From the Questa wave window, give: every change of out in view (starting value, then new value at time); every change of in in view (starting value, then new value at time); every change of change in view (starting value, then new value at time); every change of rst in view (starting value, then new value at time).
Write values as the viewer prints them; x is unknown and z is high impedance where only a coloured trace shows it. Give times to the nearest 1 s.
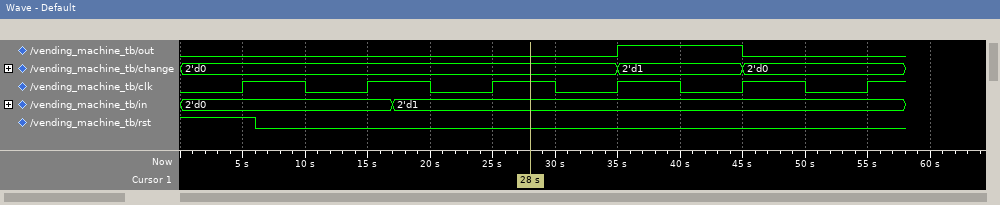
0, 1 at 35 s, 0 at 45 s
2'd0, 2'd1 at 17 s
2'd0, 2'd1 at 35 s, 2'd0 at 45 s
1, 0 at 6 s
